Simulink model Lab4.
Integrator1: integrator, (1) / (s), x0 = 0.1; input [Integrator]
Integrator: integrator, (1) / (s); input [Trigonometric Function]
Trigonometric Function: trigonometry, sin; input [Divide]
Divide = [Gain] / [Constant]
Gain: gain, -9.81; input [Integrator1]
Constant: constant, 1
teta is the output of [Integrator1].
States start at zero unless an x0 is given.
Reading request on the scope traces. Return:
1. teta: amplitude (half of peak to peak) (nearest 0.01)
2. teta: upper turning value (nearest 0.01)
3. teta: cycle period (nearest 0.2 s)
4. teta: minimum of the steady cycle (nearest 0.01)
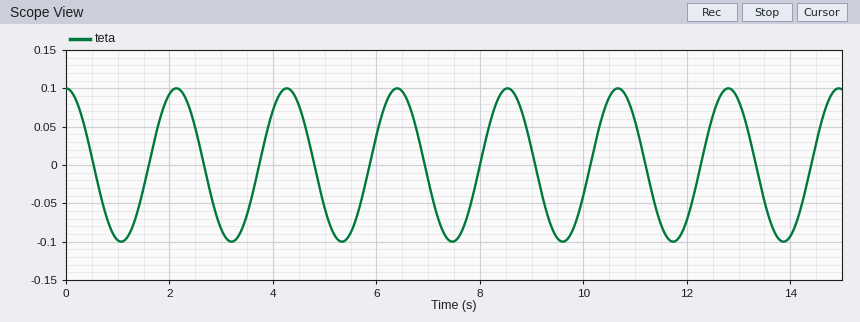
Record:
0.10
0.10
2.2 s
-0.10
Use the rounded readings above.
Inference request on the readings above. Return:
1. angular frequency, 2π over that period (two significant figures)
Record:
2.9 rad/s
